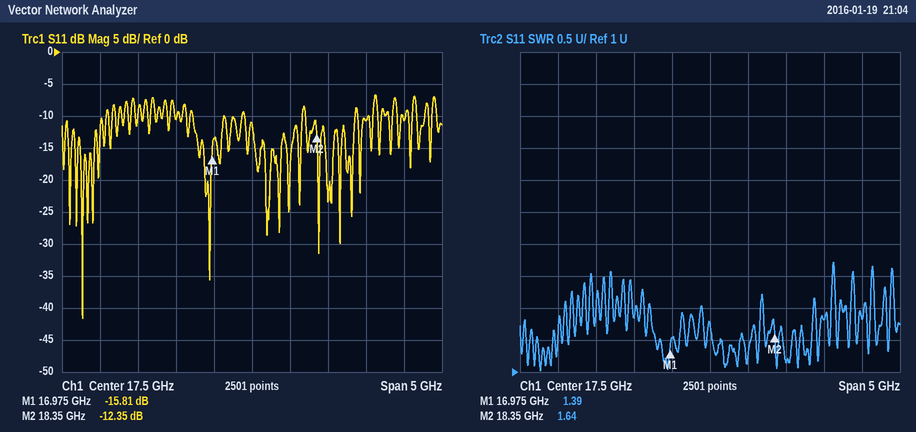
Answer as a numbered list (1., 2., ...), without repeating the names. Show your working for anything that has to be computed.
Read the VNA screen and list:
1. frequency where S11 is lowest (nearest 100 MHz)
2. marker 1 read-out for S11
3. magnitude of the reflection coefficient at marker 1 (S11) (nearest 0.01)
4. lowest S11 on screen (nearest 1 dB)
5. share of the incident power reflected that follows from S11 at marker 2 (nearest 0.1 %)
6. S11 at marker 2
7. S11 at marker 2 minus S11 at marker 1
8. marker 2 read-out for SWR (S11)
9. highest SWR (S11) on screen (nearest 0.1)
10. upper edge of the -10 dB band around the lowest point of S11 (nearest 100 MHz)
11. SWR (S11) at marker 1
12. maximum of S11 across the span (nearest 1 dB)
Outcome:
1. 15.3 GHz
2. -15.81 dB
3. 10^(-15.81/20) ≈ 0.16
4. -42 dB
5. 10^(-12.35/10) ≈ 5.8 %
6. -12.35 dB
7. -12.35 − (-15.81) = 3.46 dB
8. 1.64
9. 2.7
10. 15.6 GHz
11. 1.39
12. -7 dB
